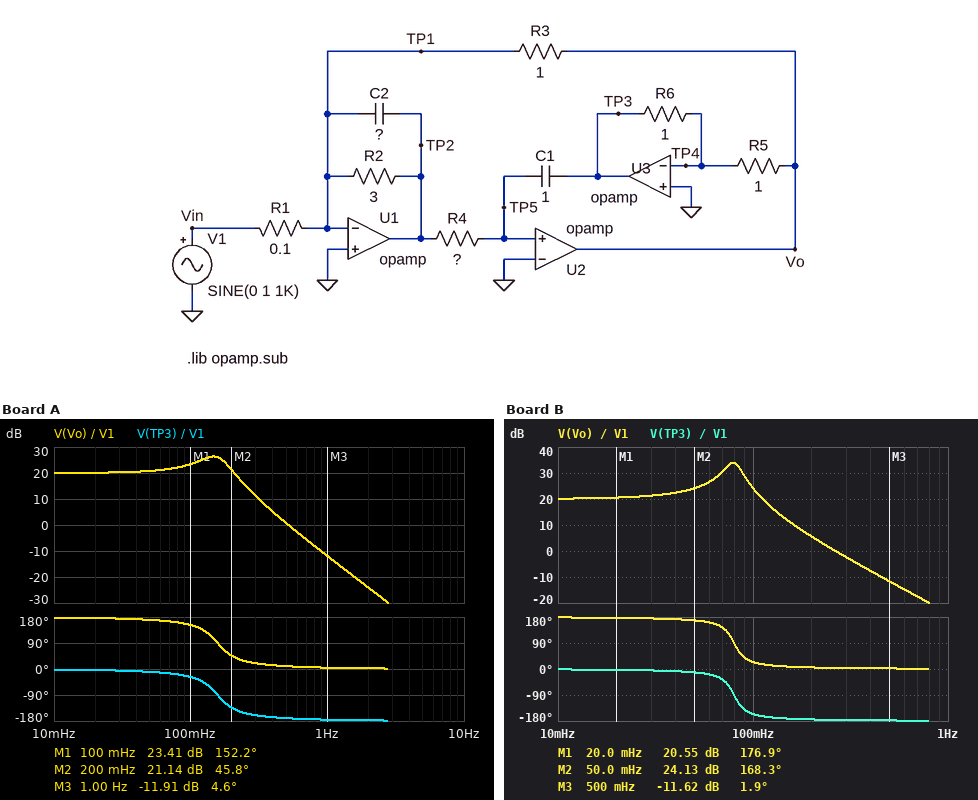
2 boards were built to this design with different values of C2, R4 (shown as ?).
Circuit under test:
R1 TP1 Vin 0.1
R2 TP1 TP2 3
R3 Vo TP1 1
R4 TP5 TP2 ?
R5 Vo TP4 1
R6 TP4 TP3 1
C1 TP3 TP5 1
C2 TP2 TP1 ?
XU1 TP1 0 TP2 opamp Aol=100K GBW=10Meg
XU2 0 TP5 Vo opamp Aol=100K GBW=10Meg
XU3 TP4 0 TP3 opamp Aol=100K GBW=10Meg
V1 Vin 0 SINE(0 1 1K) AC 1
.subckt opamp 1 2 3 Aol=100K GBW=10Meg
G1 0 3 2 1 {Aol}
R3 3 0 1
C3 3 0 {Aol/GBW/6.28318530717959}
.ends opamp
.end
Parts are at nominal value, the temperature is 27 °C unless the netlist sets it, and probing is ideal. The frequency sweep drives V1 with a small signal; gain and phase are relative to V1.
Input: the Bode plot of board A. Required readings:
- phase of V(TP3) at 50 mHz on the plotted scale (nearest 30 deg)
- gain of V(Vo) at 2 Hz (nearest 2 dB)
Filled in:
0 deg
-24 dB
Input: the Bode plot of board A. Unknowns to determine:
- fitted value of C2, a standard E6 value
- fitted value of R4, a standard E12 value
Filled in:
680 mF
1.5 Ω
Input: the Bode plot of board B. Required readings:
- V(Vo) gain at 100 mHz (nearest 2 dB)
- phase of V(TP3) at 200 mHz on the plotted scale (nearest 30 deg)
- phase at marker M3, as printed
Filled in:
24 dB
-180 deg
1.9 deg
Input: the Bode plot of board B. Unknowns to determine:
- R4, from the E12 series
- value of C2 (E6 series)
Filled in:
1.2 Ω
3.3 F
